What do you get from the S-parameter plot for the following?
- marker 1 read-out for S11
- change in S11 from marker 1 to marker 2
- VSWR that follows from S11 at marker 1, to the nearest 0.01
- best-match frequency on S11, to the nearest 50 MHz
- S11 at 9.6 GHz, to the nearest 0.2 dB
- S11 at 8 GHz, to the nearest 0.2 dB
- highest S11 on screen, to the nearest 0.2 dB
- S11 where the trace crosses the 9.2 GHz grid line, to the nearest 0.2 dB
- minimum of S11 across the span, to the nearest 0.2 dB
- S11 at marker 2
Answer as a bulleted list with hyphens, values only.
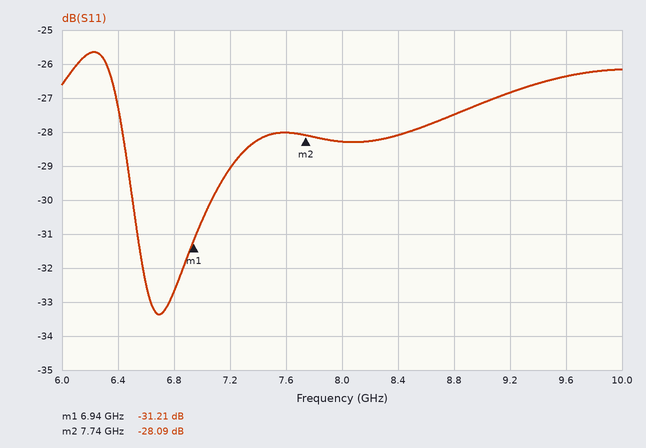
- -31.21 dB
- 3.12 dB
- 1.06
- 6.70 GHz
- -26.4 dB
- -28.2 dB
- -25.6 dB
- -26.8 dB
- -33.4 dB
- -28.09 dB
